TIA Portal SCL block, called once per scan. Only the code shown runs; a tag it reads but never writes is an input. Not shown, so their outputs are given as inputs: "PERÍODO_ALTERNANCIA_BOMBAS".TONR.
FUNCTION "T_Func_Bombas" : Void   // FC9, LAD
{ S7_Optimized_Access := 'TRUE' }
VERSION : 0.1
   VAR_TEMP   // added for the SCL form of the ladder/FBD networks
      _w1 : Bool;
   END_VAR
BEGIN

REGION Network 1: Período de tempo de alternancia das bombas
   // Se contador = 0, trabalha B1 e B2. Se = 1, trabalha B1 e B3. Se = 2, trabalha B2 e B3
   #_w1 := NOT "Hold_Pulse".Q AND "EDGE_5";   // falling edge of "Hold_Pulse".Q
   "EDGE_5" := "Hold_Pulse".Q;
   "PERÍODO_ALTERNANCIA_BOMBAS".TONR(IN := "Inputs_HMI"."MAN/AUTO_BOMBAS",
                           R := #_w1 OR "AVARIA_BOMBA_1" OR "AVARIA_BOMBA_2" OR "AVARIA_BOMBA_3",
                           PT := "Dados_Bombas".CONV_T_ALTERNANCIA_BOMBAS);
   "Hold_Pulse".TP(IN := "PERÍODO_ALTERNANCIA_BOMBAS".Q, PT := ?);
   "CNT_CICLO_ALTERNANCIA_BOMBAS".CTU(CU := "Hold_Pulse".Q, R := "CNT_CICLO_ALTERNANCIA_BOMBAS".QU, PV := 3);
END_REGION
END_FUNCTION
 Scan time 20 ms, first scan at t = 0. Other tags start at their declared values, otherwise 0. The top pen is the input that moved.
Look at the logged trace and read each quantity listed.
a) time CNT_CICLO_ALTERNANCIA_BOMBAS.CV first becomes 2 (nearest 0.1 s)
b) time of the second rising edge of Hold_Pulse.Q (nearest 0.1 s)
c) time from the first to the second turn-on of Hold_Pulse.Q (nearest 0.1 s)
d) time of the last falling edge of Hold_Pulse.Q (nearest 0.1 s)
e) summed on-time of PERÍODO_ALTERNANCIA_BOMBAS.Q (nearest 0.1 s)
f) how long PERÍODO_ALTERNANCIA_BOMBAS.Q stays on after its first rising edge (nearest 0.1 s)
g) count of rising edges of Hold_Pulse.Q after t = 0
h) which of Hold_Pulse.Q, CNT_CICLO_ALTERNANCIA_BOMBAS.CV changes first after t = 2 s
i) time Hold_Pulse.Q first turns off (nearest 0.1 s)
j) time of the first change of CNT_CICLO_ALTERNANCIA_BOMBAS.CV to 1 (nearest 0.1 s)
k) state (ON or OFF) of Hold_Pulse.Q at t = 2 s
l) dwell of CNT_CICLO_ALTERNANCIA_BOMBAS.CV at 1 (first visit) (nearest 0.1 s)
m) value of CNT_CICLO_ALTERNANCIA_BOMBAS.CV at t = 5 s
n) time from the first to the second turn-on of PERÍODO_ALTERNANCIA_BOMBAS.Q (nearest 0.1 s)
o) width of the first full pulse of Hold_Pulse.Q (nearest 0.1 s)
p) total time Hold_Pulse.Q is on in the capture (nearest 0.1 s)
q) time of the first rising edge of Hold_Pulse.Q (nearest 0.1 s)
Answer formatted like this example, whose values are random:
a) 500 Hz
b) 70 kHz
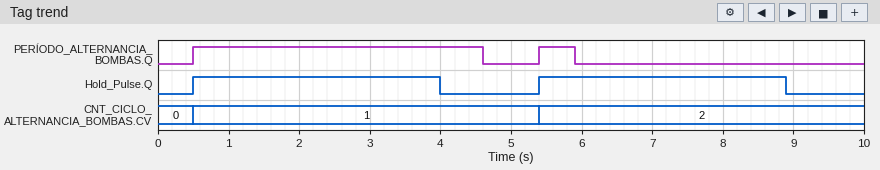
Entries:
a) 5.4 s
b) 5.4 s
c) 4.9 s
d) 8.9 s
e) 4.6 s
f) 4.1 s
g) 2
h) Hold_Pulse.Q
i) 4.0 s
j) 0.5 s
k) ON
l) 4.9 s
m) 1
n) 4.9 s
o) 3.5 s
p) 7.0 s
q) 0.5 s
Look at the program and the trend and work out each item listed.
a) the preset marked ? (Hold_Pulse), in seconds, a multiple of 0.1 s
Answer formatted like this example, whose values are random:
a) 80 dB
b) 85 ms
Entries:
a) 3.5 s
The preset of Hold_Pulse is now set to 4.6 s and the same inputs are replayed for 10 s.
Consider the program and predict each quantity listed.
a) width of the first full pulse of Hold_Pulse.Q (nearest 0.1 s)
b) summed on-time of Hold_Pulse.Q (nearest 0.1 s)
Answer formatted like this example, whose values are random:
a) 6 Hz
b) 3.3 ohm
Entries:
a) 4.6 s
b) 9.2 s
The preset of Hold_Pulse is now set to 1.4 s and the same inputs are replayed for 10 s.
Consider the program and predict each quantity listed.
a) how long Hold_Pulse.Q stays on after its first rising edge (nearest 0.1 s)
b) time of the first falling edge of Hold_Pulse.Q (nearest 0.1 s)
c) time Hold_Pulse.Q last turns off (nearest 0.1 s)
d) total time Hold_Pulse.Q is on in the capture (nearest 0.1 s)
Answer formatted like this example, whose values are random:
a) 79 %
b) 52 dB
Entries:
a) 1.4 s
b) 1.9 s
c) 6.8 s
d) 2.8 s
